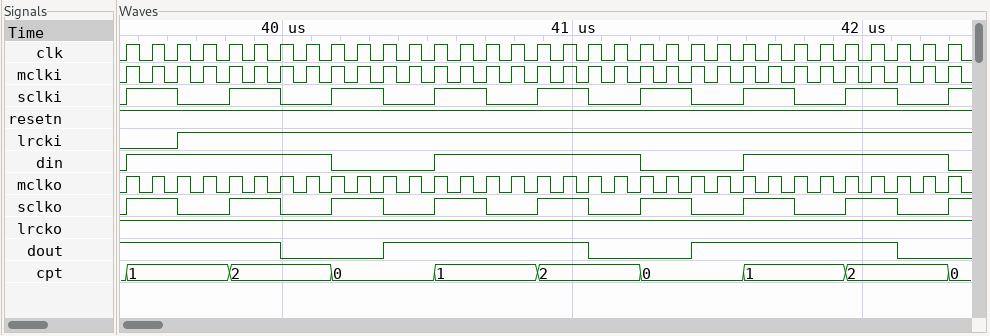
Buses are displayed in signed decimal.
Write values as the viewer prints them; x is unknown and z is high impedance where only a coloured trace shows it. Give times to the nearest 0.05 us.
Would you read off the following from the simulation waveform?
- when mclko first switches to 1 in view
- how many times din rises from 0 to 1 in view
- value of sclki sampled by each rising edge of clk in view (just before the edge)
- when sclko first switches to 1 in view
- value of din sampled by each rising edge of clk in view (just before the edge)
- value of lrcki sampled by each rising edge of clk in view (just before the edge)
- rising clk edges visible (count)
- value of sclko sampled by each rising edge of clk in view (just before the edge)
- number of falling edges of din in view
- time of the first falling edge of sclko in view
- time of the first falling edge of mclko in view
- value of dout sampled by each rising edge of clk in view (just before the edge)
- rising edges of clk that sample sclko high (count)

39.45 us
3
0 1 1 0 0 1 1 0 0 1 1 0 0 1 1 0 0 1 1 0 0 1 1 0 0 1 1 0 0 1 1 0 0
39.45 us
0 1 1 1 1 1 1 1 1 0 0 0 0 1 1 1 1 1 1 1 1 0 0 0 0 1 1 1 1 1 1 1 1
0 0 0 1 1 1 1 1 1 1 1 1 1 1 1 1 1 1 1 1 1 1 1 1 1 1 1 1 1 1 1 1 1
33
0 1 1 0 0 1 1 0 0 1 1 0 0 1 1 0 0 1 1 0 0 1 1 0 0 1 1 0 0 1 1 0 0
3
39.65 us
39.5 us
1 1 1 1 1 1 1 0 0 0 0 1 1 1 1 1 1 1 1 0 0 0 0 1 1 1 1 1 1 1 1 0 0
16
